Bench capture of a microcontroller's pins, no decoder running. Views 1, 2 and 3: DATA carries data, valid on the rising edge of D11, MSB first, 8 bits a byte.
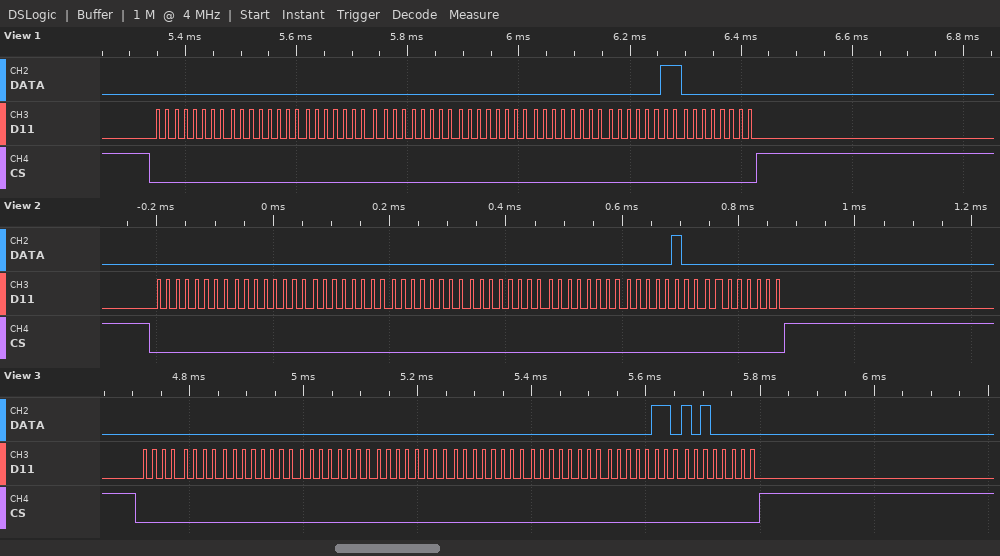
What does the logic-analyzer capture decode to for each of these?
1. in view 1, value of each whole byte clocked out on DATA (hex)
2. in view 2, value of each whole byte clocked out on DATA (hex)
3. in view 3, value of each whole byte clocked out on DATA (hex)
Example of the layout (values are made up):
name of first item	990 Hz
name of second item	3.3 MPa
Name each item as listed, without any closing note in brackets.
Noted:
in view 1, value of each whole byte clocked out on DATA	0x00 0x00 0x00 0x00 0x00 0x00 0x03 0x00
in view 2, value of each whole byte clocked out on DATA	00 00 00 00 00 00 04 00
in view 3, value of each whole byte clocked out on DATA	00 00 00 00 00 00 06 A0
